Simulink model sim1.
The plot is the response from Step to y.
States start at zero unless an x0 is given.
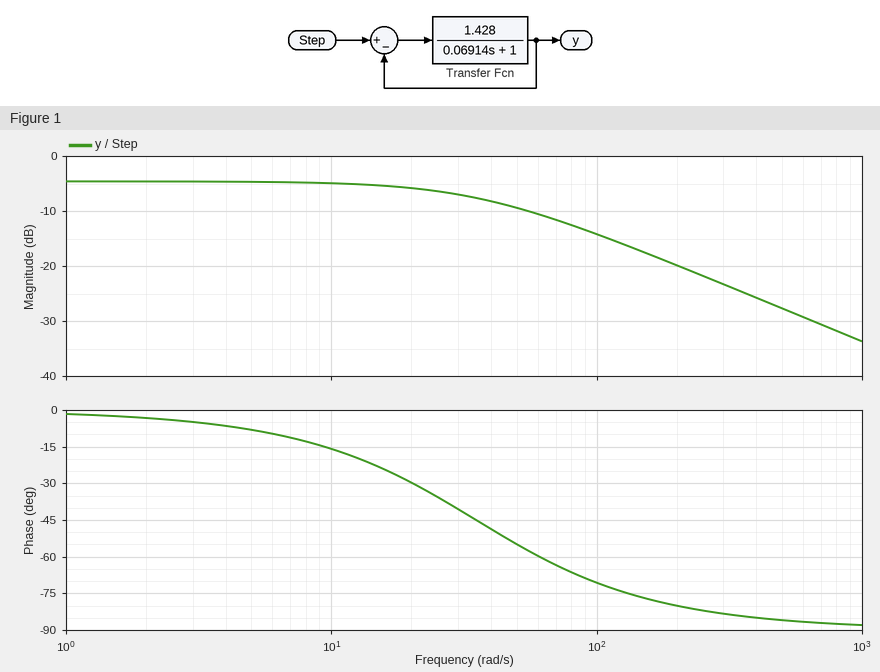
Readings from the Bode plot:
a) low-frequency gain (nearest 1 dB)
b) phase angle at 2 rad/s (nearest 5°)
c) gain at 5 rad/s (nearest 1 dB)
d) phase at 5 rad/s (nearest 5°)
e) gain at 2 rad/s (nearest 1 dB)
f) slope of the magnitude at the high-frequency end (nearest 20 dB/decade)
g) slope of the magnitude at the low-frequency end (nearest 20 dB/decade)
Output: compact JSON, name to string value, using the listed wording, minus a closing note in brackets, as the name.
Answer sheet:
{"low-frequency gain": "-5 dB", "phase angle at 2 rad/s": "-5°", "gain at 5 rad/s": "-5 dB", "phase at 5 rad/s": "-10°", "gain at 2 rad/s": "-5 dB", "slope of the magnitude at the high-frequency end": "-20 dB/decade", "slope of the magnitude at the low-frequency end": "0 dB/decade"}
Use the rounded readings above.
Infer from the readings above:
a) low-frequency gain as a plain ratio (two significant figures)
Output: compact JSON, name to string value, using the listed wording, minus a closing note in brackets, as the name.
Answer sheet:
{"low-frequency gain as a plain ratio": "0.56"}
